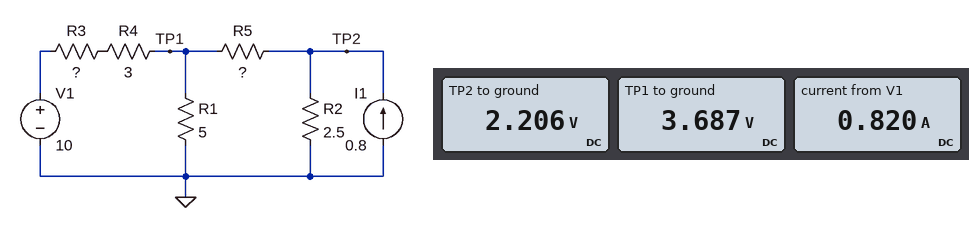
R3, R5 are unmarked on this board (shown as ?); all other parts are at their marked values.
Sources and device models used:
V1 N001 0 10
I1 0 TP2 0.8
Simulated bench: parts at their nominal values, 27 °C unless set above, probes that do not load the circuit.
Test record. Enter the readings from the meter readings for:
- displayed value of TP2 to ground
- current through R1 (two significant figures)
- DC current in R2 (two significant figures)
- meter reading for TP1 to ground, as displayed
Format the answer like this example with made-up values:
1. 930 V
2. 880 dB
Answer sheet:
1. 2.206 V
2. 740 mA
3. 880 mA
4. 3.687 V
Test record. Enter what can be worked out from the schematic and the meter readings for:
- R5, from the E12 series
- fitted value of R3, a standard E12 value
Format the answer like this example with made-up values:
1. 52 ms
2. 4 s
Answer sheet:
1. 18 Ω
2. 4.7 Ω
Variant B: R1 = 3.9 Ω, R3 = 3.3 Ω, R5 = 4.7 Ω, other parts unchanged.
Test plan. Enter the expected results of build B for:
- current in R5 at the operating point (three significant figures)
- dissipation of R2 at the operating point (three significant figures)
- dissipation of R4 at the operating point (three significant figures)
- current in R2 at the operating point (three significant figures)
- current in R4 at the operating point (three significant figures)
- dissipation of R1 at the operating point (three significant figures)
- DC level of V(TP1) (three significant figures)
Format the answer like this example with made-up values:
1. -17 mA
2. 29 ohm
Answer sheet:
1. 190 mA
2. 2.45 W
3. 3.33 W
4. 990 mA
5. 1.05 A
6. 2.91 W
7. 3.37 V
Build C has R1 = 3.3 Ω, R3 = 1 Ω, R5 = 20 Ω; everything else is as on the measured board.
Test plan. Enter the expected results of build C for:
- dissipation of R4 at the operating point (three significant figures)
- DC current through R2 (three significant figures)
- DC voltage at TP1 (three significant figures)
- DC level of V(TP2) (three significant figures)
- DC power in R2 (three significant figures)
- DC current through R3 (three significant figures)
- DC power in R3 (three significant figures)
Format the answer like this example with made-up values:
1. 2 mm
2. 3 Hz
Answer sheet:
1. 6.02 W
2. 904 mA
3. 4.33 V
4. 2.26 V
5. 2.04 W
6. 1.42 A
7. 2.01 W
